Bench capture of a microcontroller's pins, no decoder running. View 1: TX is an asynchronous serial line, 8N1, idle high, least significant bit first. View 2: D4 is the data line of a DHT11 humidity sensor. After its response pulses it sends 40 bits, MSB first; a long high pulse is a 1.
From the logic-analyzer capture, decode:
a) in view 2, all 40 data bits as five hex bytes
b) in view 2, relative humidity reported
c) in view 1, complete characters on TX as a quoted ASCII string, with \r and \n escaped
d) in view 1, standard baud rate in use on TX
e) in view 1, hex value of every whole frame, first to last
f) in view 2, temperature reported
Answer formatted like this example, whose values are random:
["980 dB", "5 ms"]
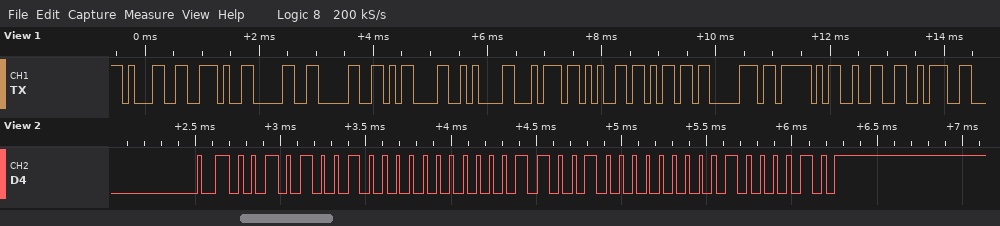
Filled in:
["29 00 19 00 42", "41 %", "\"1.00\\r\\ntemp_2:\"", "9600 baud", "31 2E 30 30 0D 0A 74 65 6D 70 5F 32 3A", "25.0 °C"]
